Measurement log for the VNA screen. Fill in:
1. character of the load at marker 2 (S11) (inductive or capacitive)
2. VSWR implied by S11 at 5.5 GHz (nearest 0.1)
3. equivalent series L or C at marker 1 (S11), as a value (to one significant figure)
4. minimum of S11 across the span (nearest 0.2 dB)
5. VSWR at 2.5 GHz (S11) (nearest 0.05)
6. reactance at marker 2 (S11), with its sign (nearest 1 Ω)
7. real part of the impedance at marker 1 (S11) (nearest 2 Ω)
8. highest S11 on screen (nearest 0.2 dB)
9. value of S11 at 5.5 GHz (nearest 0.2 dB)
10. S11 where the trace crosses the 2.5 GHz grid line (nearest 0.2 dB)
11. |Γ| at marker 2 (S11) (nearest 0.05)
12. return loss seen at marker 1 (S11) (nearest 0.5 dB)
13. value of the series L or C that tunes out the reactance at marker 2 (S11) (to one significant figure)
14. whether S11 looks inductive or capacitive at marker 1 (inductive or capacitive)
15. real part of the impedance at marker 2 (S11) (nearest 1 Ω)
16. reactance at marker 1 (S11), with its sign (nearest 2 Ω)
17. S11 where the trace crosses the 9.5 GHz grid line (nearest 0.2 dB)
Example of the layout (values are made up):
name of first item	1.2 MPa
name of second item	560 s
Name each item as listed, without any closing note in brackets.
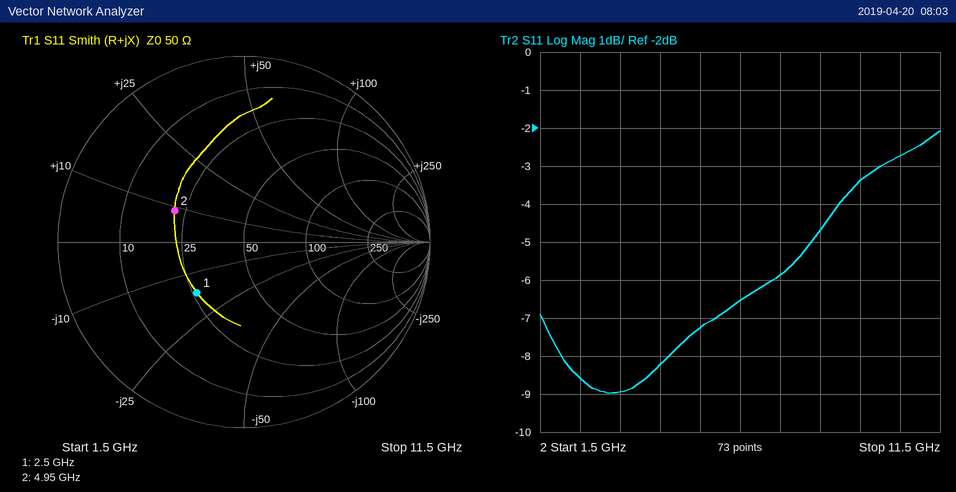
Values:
character of the load at marker 2 (S11)	inductive
VSWR implied by S11 at 5.5 GHz	2.5
equivalent series L or C at marker 1 (S11), as a value	4 pF
minimum of S11 across the span	-9.0 dB
VSWR at 2.5 GHz (S11)	2.20
reactance at marker 2 (S11), with its sign	+9 Ω
real part of the impedance at marker 1 (S11)	26 Ω
highest S11 on screen	-2.0 dB
value of S11 at 5.5 GHz	-7.2 dB
S11 where the trace crosses the 2.5 GHz grid line	-8.6 dB
|Γ| at marker 2 (S11)	0.40
return loss seen at marker 1 (S11)	8.5 dB
value of the series L or C that tunes out the reactance at marker 2 (S11)	4 pF
whether S11 looks inductive or capacitive at marker 1	capacitive
real part of the impedance at marker 2 (S11)	22 Ω
reactance at marker 1 (S11), with its sign	-16 Ω
S11 where the trace crosses the 9.5 GHz grid line	-3.4 dB
